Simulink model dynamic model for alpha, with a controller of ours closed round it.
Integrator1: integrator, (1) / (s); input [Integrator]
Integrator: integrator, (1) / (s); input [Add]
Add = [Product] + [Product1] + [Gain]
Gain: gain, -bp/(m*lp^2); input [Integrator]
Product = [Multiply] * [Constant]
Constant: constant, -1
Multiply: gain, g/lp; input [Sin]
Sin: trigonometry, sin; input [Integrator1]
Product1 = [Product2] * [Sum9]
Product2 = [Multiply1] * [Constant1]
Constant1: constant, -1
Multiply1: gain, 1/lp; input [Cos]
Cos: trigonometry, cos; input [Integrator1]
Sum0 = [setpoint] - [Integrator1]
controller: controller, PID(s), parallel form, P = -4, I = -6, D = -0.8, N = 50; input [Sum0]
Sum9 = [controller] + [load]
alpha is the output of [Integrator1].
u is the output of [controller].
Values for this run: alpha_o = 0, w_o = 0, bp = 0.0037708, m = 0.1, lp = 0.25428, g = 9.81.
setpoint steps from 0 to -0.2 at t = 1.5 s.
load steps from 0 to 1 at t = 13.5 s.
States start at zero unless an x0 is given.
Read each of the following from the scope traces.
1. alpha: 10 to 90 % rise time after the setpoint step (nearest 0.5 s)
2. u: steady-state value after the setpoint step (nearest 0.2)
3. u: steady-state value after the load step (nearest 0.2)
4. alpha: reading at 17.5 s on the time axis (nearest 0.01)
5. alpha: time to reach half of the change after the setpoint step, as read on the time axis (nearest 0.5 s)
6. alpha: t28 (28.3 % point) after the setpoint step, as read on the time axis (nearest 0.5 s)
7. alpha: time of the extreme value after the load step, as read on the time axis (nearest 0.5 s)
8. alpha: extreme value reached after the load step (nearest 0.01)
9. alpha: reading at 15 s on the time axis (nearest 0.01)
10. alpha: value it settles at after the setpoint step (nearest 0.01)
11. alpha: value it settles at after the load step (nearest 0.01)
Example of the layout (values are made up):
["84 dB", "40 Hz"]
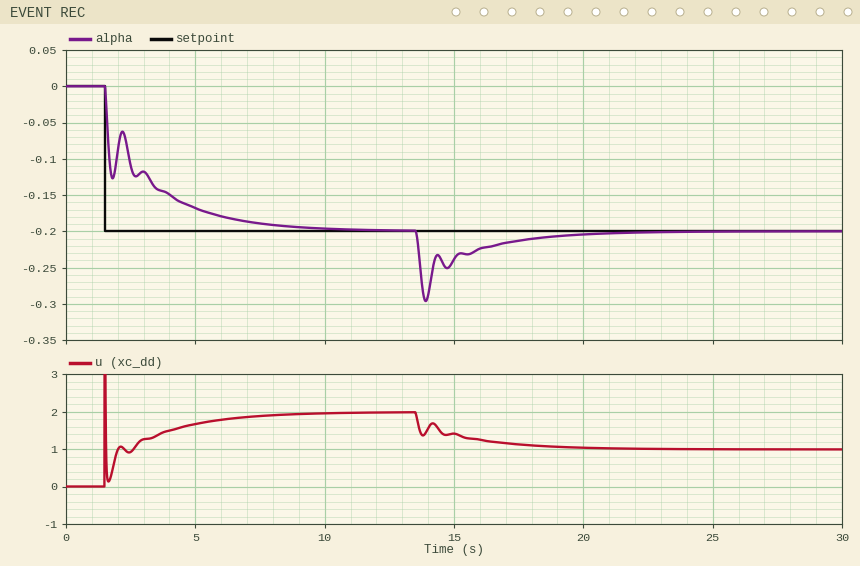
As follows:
["4.5 s", "2.0", "1.0", "-0.21", "1.5 s", "1.5 s", "14.0 s", "-0.30", "-0.24", "-0.20", "-0.20"]
